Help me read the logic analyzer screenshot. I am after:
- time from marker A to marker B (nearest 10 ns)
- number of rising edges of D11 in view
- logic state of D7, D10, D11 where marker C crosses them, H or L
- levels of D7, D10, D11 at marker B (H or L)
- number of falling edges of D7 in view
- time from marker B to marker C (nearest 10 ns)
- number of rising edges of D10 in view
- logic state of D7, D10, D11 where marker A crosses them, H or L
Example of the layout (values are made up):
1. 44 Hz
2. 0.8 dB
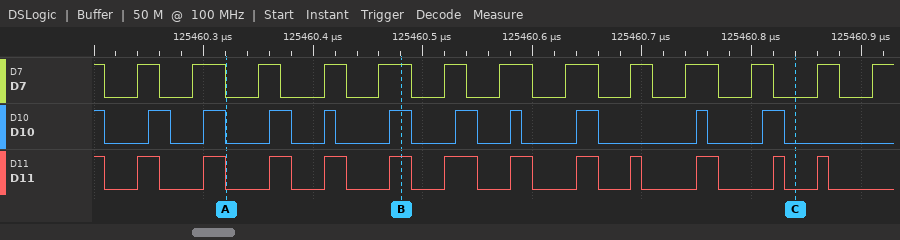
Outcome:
1. 160 ns
2. 12
3. D7=L, D10=L, D11=L
4. D7=H, D10=H, D11=H
5. 13
6. 360 ns
7. 10
8. D7=L, D10=L, D11=L
